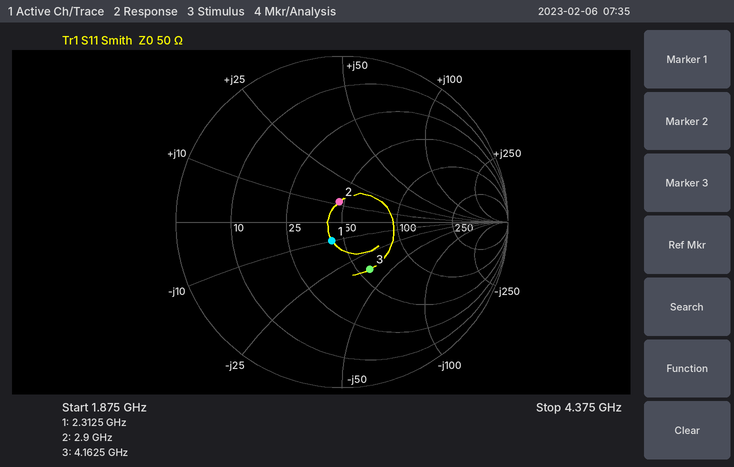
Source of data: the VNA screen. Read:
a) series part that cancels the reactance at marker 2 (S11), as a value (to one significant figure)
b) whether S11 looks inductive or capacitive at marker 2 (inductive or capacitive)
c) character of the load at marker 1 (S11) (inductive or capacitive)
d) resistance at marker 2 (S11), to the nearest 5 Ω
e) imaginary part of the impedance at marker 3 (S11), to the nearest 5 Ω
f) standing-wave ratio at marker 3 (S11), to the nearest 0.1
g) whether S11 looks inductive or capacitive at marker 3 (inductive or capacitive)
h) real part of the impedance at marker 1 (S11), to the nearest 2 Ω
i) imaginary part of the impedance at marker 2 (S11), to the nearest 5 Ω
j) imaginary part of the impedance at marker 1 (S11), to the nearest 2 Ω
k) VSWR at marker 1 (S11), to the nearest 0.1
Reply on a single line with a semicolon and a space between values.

5 pF; inductive; capacitive; 45 Ω; -35 Ω; 2.0; capacitive; 44 Ω; +10 Ω; -10 Ω; 1.3
